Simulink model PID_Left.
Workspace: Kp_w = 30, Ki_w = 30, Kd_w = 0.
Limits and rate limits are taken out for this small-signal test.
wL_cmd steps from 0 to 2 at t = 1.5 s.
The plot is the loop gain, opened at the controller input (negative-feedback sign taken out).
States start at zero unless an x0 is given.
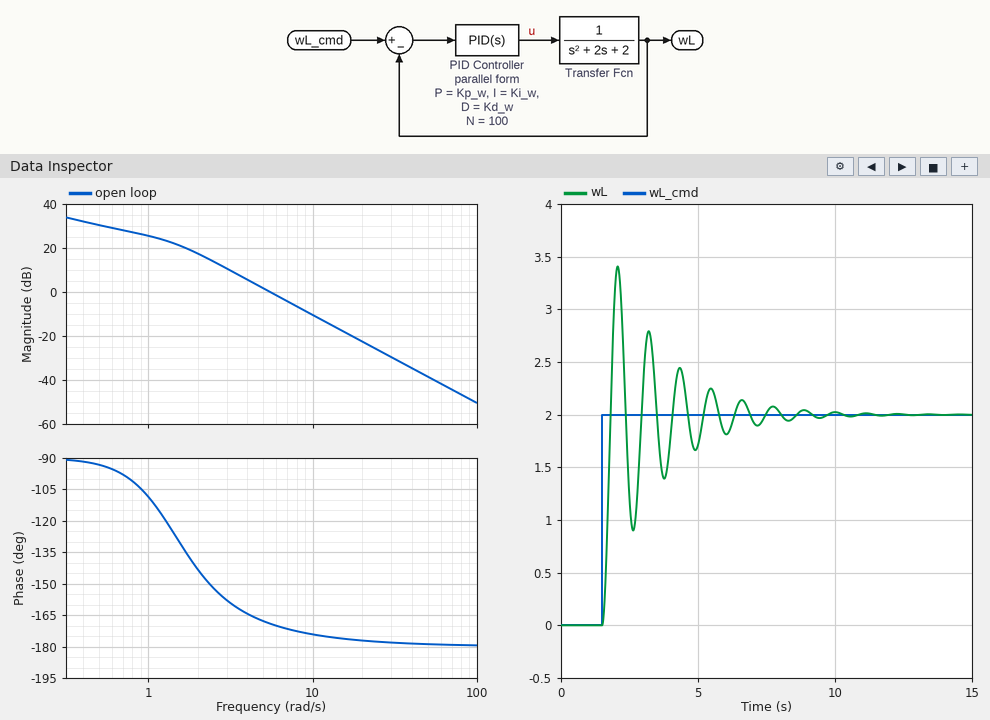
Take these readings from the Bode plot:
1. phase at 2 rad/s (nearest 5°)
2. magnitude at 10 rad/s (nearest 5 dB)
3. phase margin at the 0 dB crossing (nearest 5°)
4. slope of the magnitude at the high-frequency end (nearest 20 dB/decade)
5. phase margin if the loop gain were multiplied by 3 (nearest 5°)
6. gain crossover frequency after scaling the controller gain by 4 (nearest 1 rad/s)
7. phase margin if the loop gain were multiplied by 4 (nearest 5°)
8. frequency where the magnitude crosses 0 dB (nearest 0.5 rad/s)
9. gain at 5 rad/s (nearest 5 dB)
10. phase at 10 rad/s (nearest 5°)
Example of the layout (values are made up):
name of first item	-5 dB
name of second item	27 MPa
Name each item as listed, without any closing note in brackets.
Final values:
phase at 2 rad/s	-145°
magnitude at 10 rad/s	-10 dB
phase margin at the 0 dB crossing	10°
slope of the magnitude at the high-frequency end	-40 dB/decade
phase margin if the loop gain were multiplied by 3	5°
gain crossover frequency after scaling the controller gain by 4	11 rad/s
phase margin if the loop gain were multiplied by 4	5°
frequency where the magnitude crosses 0 dB	5.5 rad/s
gain at 5 rad/s	0 dB
phase at 10 rad/s	-175°
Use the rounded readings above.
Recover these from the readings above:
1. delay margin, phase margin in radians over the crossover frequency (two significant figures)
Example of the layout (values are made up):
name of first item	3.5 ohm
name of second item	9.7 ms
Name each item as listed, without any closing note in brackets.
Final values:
delay margin, phase margin in radians over the crossover frequency	0.032 s
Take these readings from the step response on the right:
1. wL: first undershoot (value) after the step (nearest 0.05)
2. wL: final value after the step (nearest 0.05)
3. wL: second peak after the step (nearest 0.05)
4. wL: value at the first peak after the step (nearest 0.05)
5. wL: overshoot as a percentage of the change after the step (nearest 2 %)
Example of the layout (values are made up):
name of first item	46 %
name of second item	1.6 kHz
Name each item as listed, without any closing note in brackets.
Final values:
wL: first undershoot (value) after the step	0.90
wL: final value after the step	2.00
wL: second peak after the step	2.80
wL: value at the first peak after the step	3.40
wL: overshoot as a percentage of the change after the step	70 %
